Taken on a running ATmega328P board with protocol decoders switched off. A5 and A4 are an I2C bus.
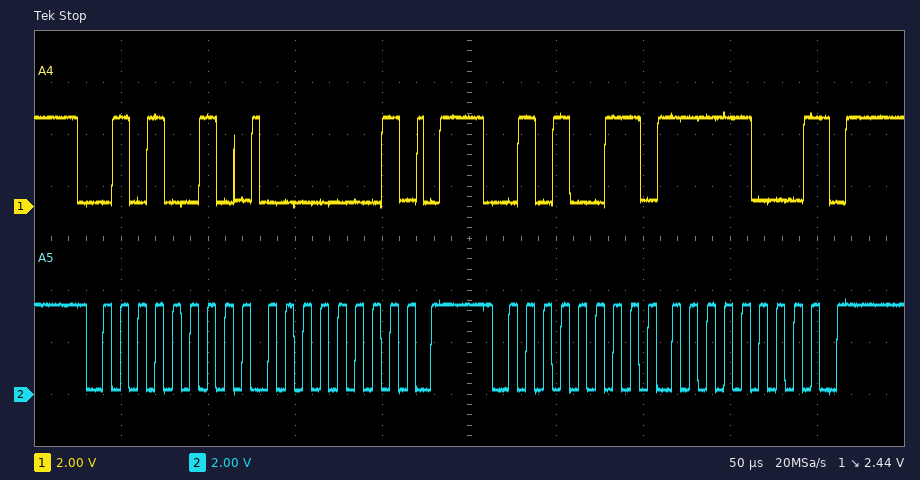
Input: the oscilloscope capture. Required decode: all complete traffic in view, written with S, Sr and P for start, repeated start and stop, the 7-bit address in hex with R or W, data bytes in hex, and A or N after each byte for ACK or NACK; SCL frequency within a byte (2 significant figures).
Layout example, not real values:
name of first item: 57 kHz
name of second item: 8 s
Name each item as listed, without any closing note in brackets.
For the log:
all complete traffic in view, written with S, Sr and P for start, repeated start and stop, the 7-bit address in hex with R or W, data bytes in hex, and A or N after each byte for ACK or NACK: S 29W A 01 A P S 29R A F8 N P
SCL frequency within a byte: 100 kHz
